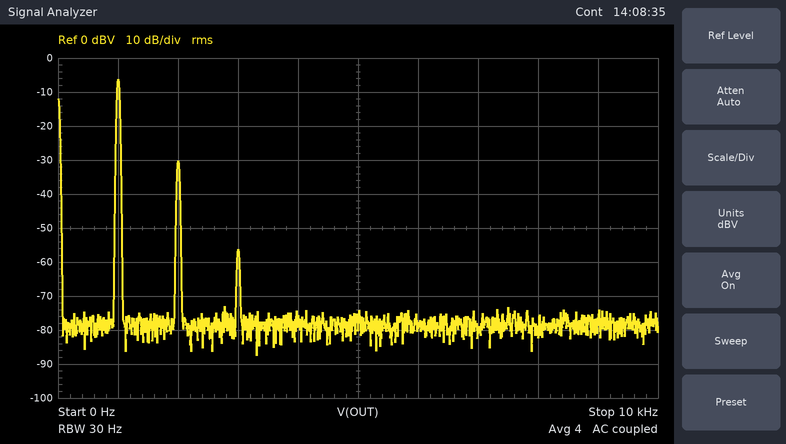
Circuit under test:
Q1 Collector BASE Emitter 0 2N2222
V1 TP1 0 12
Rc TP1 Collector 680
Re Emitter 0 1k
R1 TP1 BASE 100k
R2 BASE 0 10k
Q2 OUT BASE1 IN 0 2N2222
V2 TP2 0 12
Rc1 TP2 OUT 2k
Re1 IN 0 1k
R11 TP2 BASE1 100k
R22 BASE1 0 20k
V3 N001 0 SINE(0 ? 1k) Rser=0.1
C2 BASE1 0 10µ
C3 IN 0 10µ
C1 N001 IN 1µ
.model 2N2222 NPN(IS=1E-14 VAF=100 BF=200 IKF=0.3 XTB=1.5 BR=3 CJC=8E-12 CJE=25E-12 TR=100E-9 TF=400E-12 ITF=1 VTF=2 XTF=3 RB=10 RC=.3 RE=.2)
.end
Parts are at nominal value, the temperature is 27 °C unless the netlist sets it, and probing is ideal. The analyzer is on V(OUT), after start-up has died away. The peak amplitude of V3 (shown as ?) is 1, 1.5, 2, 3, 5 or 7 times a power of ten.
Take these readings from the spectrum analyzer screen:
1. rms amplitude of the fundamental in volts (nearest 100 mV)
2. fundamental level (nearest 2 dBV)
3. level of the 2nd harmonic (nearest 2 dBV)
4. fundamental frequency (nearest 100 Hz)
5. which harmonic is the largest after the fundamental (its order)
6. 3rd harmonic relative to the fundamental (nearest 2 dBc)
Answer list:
500 mV
-6 dBV
-30 dBV
1.0 kHz
2
-50 dBc
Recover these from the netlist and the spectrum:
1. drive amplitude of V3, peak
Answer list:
100 mV
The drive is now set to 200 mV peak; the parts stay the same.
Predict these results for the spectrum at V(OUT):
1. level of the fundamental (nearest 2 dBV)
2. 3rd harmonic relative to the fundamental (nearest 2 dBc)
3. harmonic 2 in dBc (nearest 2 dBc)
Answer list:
0 dBV
-38 dBc
-18 dBc
